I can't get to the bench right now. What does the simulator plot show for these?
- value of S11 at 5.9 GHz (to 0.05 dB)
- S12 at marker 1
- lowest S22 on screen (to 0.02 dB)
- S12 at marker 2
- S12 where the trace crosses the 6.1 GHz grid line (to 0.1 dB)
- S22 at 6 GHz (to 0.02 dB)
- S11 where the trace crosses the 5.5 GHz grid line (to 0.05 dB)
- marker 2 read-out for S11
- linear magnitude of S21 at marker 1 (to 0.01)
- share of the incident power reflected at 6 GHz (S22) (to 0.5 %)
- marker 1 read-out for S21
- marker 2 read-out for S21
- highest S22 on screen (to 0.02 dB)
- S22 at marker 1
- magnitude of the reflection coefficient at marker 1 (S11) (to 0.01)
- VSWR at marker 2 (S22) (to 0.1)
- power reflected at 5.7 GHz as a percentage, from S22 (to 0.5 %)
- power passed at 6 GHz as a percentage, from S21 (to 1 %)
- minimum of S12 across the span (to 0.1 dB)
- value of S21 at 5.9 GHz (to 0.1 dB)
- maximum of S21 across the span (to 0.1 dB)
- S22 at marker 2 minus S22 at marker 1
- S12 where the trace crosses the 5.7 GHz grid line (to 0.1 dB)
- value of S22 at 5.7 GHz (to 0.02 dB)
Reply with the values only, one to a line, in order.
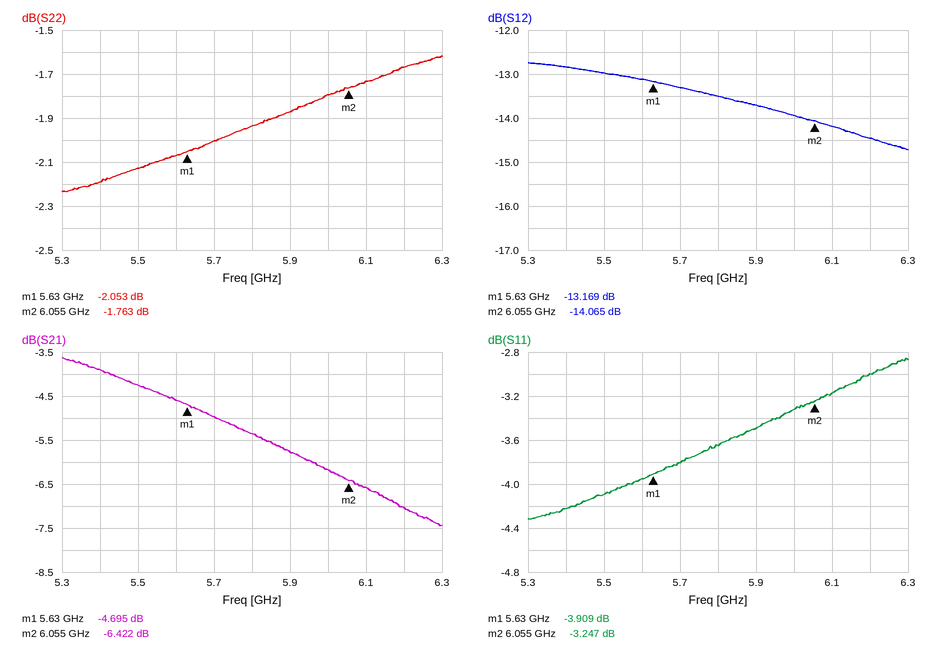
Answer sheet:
-3.50 dB
-13.169 dB
-2.24 dB
-14.065 dB
-14.2 dB
-1.80 dB
-4.10 dB
-3.247 dB
0.58
66.0 %
-4.695 dB
-6.422 dB
-1.62 dB
-2.053 dB
0.64
9.9
63.0 %
24 %
-14.7 dB
-5.8 dB
-3.6 dB
0.290 dB
-13.3 dB
-2.00 dB
